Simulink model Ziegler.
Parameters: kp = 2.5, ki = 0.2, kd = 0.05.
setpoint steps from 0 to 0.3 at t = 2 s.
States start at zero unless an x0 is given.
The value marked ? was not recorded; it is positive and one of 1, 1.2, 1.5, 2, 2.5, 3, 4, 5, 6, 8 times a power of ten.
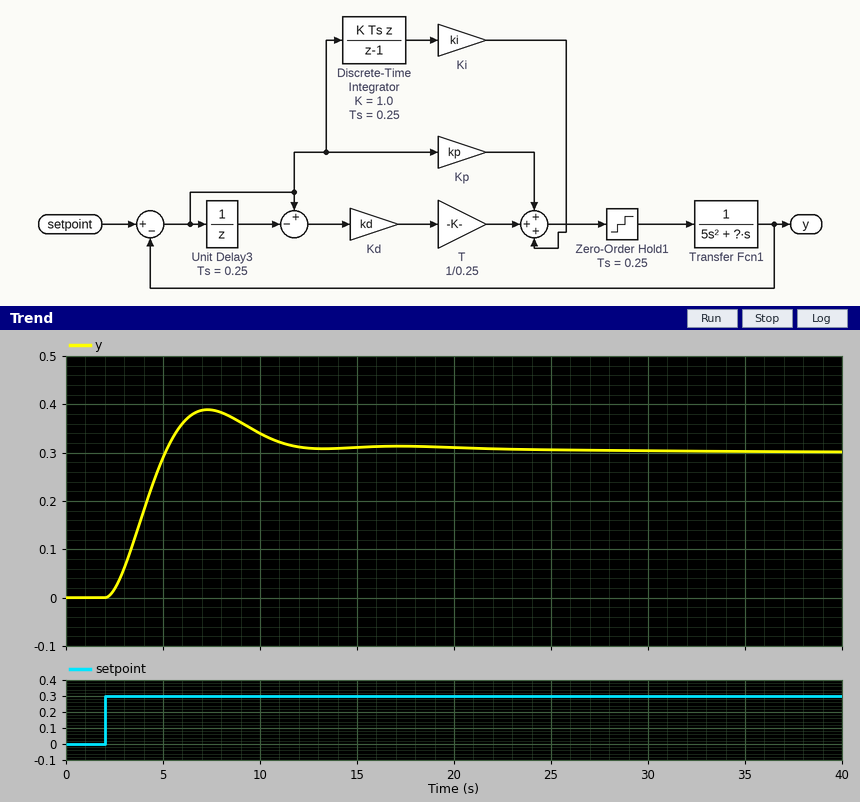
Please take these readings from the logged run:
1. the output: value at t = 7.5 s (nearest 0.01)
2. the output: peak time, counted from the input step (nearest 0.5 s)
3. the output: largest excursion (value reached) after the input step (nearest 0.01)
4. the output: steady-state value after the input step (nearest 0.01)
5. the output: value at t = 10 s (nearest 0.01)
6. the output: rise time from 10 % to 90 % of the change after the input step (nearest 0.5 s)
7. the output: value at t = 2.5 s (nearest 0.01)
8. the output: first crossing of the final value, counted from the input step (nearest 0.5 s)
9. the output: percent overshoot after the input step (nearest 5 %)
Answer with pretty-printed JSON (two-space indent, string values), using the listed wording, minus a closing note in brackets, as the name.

{
  "the output: value at t = 7.5 s": "0.39",
  "the output: peak time, counted from the input step": "5.5 s",
  "the output: largest excursion (value reached) after the input step": "0.39",
  "the output: steady-state value after the input step": "0.30",
  "the output: value at t = 10 s": "0.34",
  "the output: rise time from 10 % to 90 % of the change after the input step": "2.0 s",
  "the output: value at t = 2.5 s": "0.02",
  "the output: first crossing of the final value, counted from the input step": "3.0 s",
  "the output: percent overshoot after the input step": "30 %"
}
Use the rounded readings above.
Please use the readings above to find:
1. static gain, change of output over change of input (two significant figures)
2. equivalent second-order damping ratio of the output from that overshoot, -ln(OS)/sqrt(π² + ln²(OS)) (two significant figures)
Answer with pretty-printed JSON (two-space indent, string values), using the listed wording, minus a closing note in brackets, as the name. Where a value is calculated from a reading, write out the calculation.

{
  "static gain, change of output over change of input": "(0.3 - 0) / (0.3 - 0) = 1.0",
  "equivalent second-order damping ratio of the output from that overshoot, -ln(OS)/sqrt(π² + ln²(OS))": "ln(0.3) = -1.204; 1.204 / sqrt(9.870 + 1.450) = 0.36"
}
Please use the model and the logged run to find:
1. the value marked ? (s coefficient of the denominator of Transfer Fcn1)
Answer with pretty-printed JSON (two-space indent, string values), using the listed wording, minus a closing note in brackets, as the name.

{
  "the value marked ?": "4"
}
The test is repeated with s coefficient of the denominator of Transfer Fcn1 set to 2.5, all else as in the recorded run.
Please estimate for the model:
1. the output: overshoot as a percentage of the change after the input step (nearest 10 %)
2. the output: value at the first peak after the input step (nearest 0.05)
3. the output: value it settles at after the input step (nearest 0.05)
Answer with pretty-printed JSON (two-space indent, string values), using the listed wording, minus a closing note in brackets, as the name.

{
  "the output: overshoot as a percentage of the change after the input step": "50 %",
  "the output: value at the first peak after the input step": "0.45",
  "the output: value it settles at after the input step": "0.30"
}
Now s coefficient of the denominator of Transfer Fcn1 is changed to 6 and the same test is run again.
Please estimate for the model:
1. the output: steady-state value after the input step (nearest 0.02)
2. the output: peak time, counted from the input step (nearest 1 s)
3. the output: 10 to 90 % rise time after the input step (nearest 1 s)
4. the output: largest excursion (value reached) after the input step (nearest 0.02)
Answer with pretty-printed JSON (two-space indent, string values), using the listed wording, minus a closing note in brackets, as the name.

{
  "the output: steady-state value after the input step": "0.30",
  "the output: peak time, counted from the input step": "7 s",
  "the output: 10 to 90 % rise time after the input step": "3 s",
  "the output: largest excursion (value reached) after the input step": "0.36"
}
